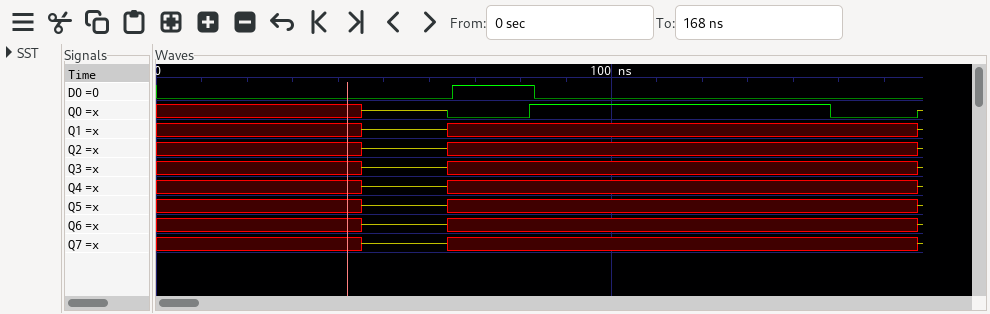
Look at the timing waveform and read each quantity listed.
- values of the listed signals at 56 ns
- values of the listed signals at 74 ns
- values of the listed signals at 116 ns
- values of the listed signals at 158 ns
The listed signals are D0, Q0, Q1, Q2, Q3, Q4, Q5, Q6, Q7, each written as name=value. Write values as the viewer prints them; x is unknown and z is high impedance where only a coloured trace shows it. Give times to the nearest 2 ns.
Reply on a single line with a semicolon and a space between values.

D0=0, Q0=z, Q1=z, Q2=z, Q3=z, Q4=z, Q5=z, Q6=z, Q7=z; D0=1, Q0=0, Q1=x, Q2=x, Q3=x, Q4=x, Q5=x, Q6=x, Q7=x; D0=0, Q0=1, Q1=x, Q2=x, Q3=x, Q4=x, Q5=x, Q6=x, Q7=x; D0=0, Q0=0, Q1=x, Q2=x, Q3=x, Q4=x, Q5=x, Q6=x, Q7=x
